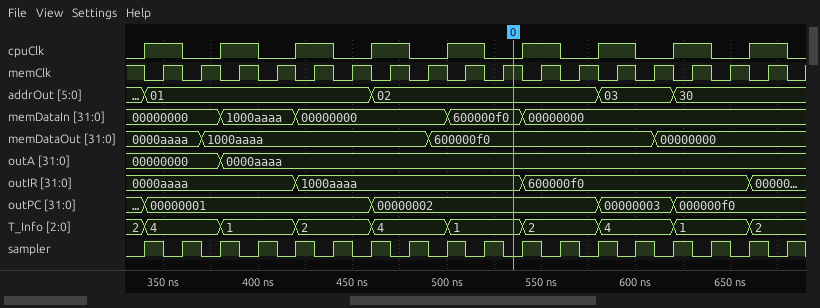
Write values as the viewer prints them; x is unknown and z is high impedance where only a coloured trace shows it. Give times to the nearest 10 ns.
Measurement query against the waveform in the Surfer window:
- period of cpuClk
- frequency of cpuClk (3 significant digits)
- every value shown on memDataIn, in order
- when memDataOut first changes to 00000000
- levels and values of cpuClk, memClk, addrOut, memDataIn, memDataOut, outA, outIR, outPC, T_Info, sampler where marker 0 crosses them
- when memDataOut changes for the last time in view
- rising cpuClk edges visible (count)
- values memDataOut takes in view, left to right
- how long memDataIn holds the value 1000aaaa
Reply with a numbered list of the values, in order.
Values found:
1. 40 ns
2. 25.0 MHz
3. 00000000, 1000aaaa, 00000000, 600000f0, 00000000
4. 610 ns
5. cpuClk=0, memClk=1, addrOut=02, memDataIn=600000f0, memDataOut=600000f0, outA=0000aaaa, outIR=1000aaaa, outPC=00000002, T_Info=1, sampler=0
6. 610 ns
7. 9
8. 0000aaaa, 1000aaaa, 600000f0, 00000000
9. 40 ns
